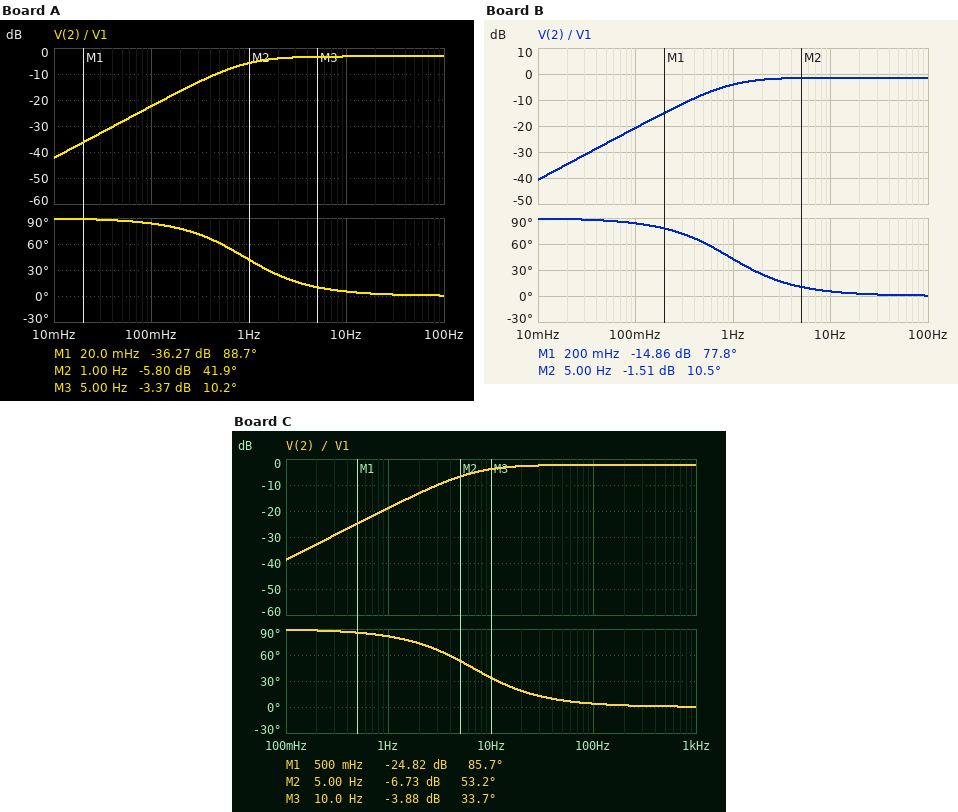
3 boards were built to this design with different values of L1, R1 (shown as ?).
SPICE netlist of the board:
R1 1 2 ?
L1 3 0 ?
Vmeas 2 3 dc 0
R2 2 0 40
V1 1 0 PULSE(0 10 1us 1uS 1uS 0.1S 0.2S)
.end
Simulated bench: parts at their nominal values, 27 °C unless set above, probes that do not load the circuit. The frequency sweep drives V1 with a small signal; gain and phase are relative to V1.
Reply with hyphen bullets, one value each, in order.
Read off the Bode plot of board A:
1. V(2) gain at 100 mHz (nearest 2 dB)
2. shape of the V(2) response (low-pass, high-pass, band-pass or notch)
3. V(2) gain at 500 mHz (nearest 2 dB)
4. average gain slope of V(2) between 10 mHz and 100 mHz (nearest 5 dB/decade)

- -22 dB
- high-pass
- -10 dB
- 20 dB/decade
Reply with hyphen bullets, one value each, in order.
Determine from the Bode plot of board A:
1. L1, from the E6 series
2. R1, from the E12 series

- 2.2 H
- 18 Ω
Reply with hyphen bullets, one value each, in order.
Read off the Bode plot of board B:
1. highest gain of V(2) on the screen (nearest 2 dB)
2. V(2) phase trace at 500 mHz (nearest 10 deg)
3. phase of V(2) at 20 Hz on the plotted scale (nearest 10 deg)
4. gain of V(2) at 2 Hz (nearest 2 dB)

- -2 dB
- 60 deg
- 0 deg
- -2 dB
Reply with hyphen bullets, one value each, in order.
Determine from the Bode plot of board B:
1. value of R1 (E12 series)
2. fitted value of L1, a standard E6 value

- 6.8 Ω
- 1 H
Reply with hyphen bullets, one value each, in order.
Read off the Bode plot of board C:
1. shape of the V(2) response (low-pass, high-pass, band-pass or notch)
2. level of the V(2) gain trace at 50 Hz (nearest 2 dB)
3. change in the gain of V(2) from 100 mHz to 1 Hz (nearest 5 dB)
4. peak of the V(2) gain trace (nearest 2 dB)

- high-pass
- -2 dB
- 20 dB
- -2 dB
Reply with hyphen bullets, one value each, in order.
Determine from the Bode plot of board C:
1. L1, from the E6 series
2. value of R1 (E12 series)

- 220 mH
- 12 Ω
